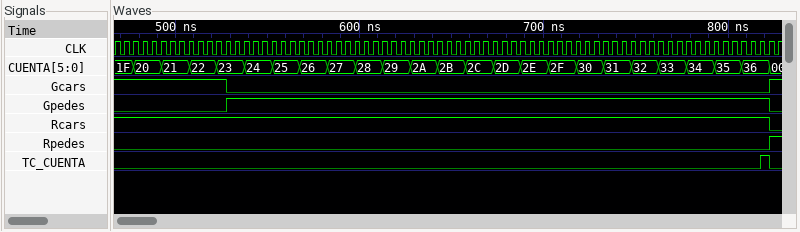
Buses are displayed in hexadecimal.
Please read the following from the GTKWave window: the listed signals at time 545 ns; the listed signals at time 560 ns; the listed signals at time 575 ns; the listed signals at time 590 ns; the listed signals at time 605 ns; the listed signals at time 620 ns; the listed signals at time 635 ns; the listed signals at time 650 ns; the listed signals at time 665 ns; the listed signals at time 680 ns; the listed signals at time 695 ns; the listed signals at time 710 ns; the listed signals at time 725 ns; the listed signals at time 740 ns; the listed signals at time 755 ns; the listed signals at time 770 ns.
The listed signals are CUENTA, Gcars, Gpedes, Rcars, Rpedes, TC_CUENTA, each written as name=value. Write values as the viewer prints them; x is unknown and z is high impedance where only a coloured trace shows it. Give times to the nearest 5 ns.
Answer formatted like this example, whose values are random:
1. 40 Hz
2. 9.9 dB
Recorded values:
1. CUENTA=24, Gcars=0, Gpedes=1, Rcars=1, Rpedes=0, TC_CUENTA=0
2. CUENTA=25, Gcars=0, Gpedes=1, Rcars=1, Rpedes=0, TC_CUENTA=0
3. CUENTA=26, Gcars=0, Gpedes=1, Rcars=1, Rpedes=0, TC_CUENTA=0
4. CUENTA=27, Gcars=0, Gpedes=1, Rcars=1, Rpedes=0, TC_CUENTA=0
5. CUENTA=28, Gcars=0, Gpedes=1, Rcars=1, Rpedes=0, TC_CUENTA=0
6. CUENTA=29, Gcars=0, Gpedes=1, Rcars=1, Rpedes=0, TC_CUENTA=0
7. CUENTA=2A, Gcars=0, Gpedes=1, Rcars=1, Rpedes=0, TC_CUENTA=0
8. CUENTA=2B, Gcars=0, Gpedes=1, Rcars=1, Rpedes=0, TC_CUENTA=0
9. CUENTA=2C, Gcars=0, Gpedes=1, Rcars=1, Rpedes=0, TC_CUENTA=0
10. CUENTA=2D, Gcars=0, Gpedes=1, Rcars=1, Rpedes=0, TC_CUENTA=0
11. CUENTA=2E, Gcars=0, Gpedes=1, Rcars=1, Rpedes=0, TC_CUENTA=0
12. CUENTA=2F, Gcars=0, Gpedes=1, Rcars=1, Rpedes=0, TC_CUENTA=0
13. CUENTA=30, Gcars=0, Gpedes=1, Rcars=1, Rpedes=0, TC_CUENTA=0
14. CUENTA=31, Gcars=0, Gpedes=1, Rcars=1, Rpedes=0, TC_CUENTA=0
15. CUENTA=32, Gcars=0, Gpedes=1, Rcars=1, Rpedes=0, TC_CUENTA=0
16. CUENTA=33, Gcars=0, Gpedes=1, Rcars=1, Rpedes=0, TC_CUENTA=0
